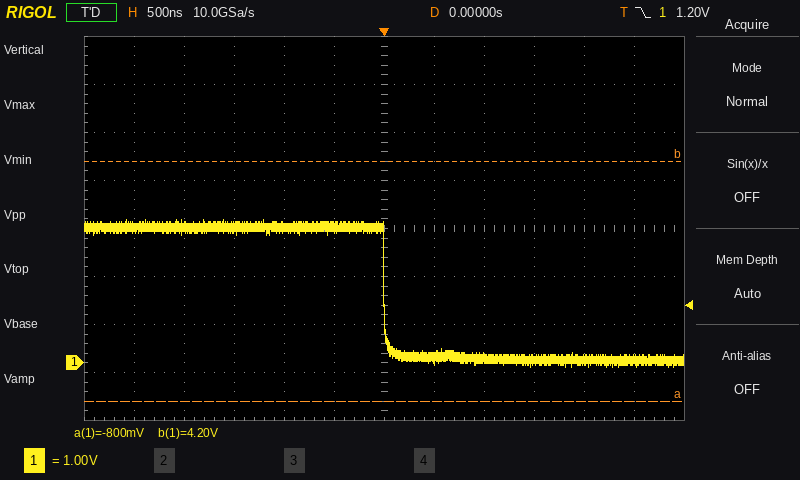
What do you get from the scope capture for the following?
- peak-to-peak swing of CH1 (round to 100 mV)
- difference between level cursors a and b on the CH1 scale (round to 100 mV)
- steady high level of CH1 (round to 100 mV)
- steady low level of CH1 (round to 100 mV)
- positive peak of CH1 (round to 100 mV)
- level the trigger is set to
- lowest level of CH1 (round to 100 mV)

3.1 V
5.0 V
2.8 V
100 mV
3.0 V
1.20 V
-100 mV
